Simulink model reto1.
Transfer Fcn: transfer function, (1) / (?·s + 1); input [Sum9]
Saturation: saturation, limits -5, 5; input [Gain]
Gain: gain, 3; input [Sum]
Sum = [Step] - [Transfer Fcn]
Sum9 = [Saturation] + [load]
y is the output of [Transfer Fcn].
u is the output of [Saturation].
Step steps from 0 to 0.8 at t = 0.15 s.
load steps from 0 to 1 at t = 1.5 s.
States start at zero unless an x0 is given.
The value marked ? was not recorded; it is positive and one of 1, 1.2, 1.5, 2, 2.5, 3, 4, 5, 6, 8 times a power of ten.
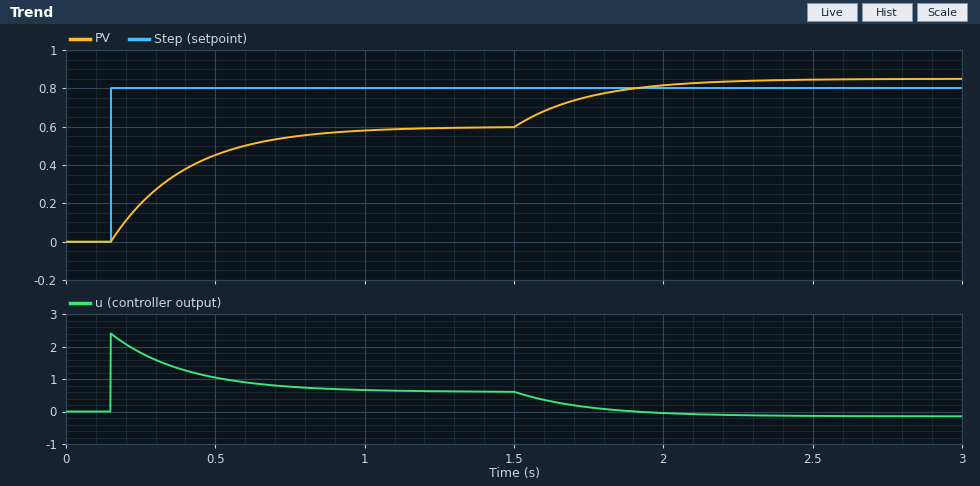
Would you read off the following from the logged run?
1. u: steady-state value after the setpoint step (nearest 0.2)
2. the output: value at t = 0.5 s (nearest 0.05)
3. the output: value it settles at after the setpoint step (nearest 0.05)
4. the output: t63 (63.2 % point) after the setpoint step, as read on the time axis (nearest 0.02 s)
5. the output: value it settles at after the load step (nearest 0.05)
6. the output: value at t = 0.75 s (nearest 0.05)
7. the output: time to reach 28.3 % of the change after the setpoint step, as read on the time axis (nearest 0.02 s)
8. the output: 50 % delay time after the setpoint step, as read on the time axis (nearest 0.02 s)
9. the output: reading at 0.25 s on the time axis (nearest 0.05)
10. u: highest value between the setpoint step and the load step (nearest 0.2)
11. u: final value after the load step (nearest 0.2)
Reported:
0.6
0.45
0.60
0.40 s
0.85
0.55
0.24 s
0.32 s
0.20
2.4
-0.2
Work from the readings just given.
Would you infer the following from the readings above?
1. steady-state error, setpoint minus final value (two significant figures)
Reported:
0.20
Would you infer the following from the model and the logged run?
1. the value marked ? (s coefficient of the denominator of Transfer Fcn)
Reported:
1
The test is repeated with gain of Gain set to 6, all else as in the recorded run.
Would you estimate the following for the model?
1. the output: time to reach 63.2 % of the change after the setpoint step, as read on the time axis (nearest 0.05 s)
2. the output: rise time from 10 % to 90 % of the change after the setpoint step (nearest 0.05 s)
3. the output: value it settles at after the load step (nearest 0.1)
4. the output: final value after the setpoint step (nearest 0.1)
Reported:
0.30 s
0.30 s
0.8
0.7
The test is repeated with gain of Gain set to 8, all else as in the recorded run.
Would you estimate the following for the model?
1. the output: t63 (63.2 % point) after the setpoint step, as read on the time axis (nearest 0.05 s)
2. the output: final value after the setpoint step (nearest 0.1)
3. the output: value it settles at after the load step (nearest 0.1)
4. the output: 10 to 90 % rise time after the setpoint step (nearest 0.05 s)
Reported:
0.25 s
0.7
0.8
0.25 s
